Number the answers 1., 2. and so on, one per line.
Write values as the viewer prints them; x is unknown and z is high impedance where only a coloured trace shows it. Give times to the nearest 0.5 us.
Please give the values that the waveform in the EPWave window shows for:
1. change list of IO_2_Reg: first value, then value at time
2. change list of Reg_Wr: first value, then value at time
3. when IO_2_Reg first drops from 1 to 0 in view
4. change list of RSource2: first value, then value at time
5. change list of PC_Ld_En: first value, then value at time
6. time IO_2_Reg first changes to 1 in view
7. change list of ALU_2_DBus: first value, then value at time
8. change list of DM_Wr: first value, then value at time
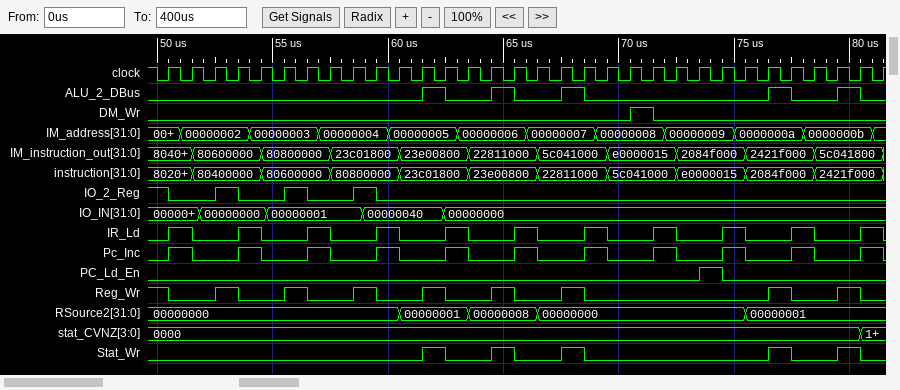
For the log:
1. 1, 0 at 50.5 us, 1 at 52.5 us, 0 at 53.5 us, 1 at 55.5 us, 0 at 56.5 us, 1 at 58.5 us, 0 at 59.5 us
2. 1, 0 at 50.5 us, 1 at 52.5 us, 0 at 53.5 us, 1 at 55.5 us, 0 at 56.5 us, 1 at 58.5 us, 0 at 59.5 us, 1 at 61.5 us, 0 at 62.5 us, 1 at 64.5 us, 0 at 65.5 us, 1 at 67.5 us, 0 at 68.5 us, 1 at 76.5 us, 0 at 77.5 us, 1 at 79.5 us, 0 at 80.5 us
3. 50.5 us
4. 00000000, 00000001 at 60.5 us, 00000008 at 63.5 us, 00000000 at 66.5 us, 00000001 at 75.5 us
5. 0, 1 at 73.5 us, 0 at 74.5 us
6. 52.5 us
7. 0, 1 at 61.5 us, 0 at 62.5 us, 1 at 64.5 us, 0 at 65.5 us, 1 at 67.5 us, 0 at 68.5 us, 1 at 76.5 us, 0 at 77.5 us, 1 at 79.5 us, 0 at 80.5 us
8. 0, 1 at 70.5 us, 0 at 71.5 us
